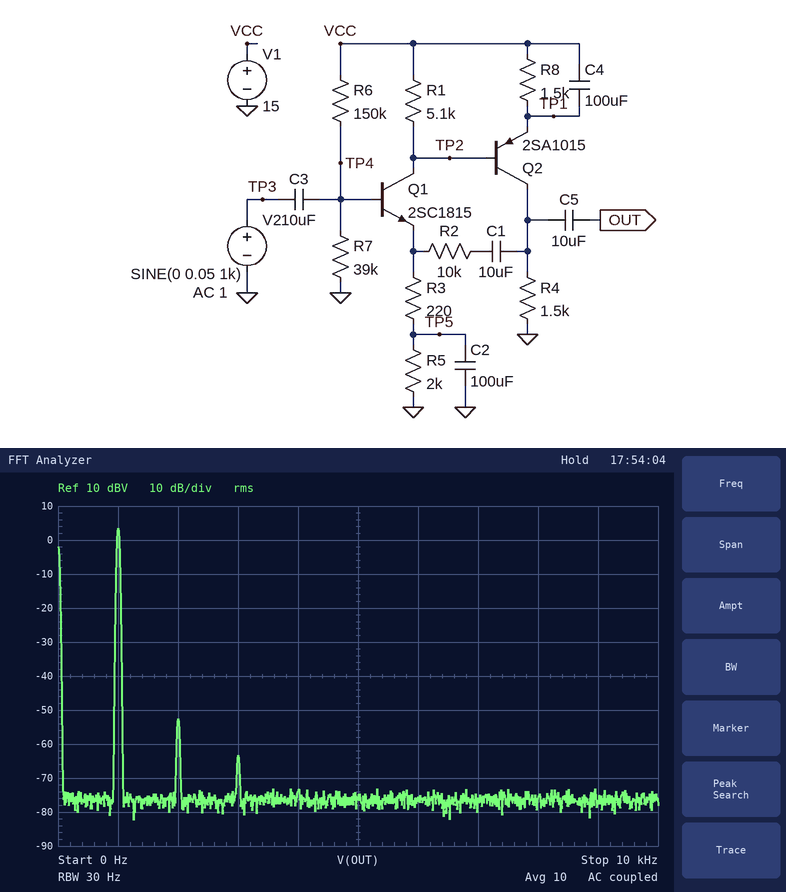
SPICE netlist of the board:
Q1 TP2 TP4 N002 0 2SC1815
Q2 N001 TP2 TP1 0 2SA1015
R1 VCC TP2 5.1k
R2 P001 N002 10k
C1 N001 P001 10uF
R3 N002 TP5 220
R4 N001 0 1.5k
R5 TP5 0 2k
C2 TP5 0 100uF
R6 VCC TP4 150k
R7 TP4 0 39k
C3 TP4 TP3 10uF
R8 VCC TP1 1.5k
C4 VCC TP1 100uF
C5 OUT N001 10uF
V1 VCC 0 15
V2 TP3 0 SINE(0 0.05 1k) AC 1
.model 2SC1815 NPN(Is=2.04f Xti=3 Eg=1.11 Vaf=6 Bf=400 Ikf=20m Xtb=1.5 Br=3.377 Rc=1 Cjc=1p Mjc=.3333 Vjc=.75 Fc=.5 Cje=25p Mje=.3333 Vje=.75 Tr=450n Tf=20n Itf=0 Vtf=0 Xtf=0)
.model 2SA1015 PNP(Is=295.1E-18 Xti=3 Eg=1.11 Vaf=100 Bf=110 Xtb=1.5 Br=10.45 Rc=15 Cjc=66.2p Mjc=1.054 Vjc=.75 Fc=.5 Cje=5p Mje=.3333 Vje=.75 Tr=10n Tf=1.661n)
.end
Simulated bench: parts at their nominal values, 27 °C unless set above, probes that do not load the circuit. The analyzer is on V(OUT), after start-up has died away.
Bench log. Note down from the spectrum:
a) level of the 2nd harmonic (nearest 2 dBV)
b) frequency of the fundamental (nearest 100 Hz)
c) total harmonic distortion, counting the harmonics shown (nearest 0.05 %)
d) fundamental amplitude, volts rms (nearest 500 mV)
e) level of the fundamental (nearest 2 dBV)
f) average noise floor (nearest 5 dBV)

-52 dBV
1.0 kHz
0.15 %
1.5 V
4 dBV
-75 dBV
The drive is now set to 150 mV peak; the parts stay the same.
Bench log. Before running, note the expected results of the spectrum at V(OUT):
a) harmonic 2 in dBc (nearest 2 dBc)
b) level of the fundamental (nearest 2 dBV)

-18 dBc
12 dBV
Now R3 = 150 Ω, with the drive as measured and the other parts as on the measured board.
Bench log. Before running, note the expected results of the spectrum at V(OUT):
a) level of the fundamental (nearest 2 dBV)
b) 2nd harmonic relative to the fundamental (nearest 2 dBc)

6 dBV
-50 dBc
